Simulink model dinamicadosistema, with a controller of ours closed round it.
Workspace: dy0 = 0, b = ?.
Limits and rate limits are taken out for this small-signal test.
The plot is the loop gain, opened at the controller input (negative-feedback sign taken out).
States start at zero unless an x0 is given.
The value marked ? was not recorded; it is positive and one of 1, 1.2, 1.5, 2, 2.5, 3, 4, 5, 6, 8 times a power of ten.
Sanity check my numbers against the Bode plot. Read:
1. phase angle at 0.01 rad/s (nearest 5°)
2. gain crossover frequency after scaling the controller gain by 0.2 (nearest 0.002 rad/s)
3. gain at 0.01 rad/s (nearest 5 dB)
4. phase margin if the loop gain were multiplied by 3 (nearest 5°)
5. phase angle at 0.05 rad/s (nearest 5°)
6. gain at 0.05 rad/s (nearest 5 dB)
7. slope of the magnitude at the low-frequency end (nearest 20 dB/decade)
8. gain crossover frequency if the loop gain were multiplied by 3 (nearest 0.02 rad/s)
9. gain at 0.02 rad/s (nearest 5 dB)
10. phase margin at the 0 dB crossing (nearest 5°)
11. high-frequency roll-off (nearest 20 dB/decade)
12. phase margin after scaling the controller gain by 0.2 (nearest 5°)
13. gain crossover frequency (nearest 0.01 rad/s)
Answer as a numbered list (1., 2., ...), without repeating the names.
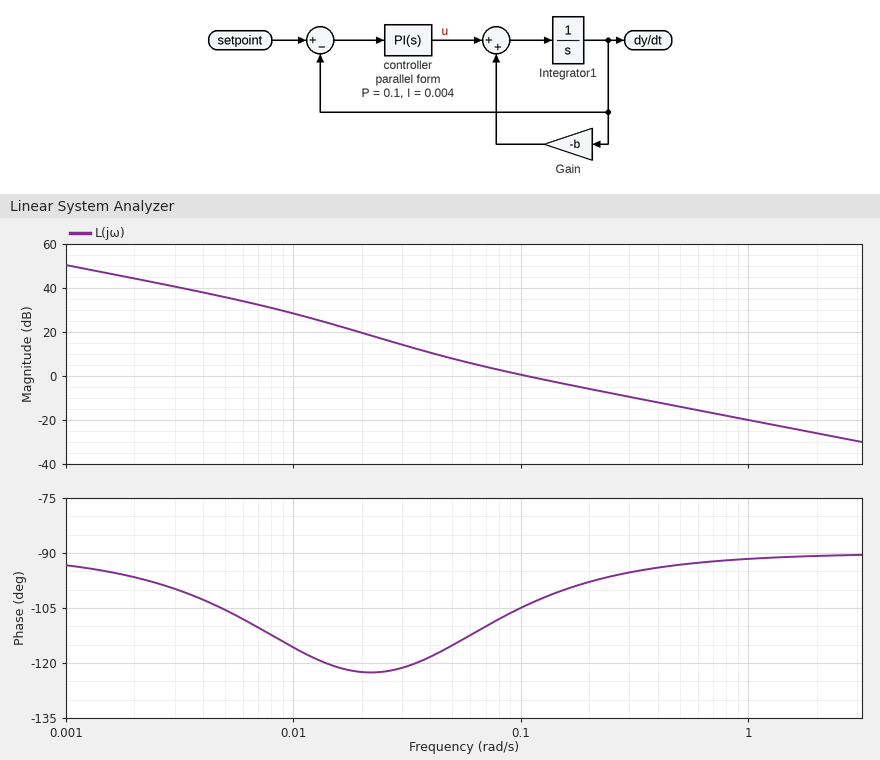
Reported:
1. -115°
2. 0.030 rad/s
3. 30 dB
4. 85°
5. -115°
6. 10 dB
7. -20 dB/decade
8. 0.30 rad/s
9. 20 dB
10. 75°
11. -20 dB/decade
12. 60°
13. 0.11 rad/s
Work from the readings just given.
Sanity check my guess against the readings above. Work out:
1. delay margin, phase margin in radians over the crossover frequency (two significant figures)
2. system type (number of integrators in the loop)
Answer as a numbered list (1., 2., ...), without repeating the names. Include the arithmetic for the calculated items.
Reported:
1. 75 × π / 180 / 0.11 = 12 s
2. 1
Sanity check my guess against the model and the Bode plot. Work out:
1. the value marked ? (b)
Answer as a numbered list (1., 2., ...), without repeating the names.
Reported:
1. 0.012
